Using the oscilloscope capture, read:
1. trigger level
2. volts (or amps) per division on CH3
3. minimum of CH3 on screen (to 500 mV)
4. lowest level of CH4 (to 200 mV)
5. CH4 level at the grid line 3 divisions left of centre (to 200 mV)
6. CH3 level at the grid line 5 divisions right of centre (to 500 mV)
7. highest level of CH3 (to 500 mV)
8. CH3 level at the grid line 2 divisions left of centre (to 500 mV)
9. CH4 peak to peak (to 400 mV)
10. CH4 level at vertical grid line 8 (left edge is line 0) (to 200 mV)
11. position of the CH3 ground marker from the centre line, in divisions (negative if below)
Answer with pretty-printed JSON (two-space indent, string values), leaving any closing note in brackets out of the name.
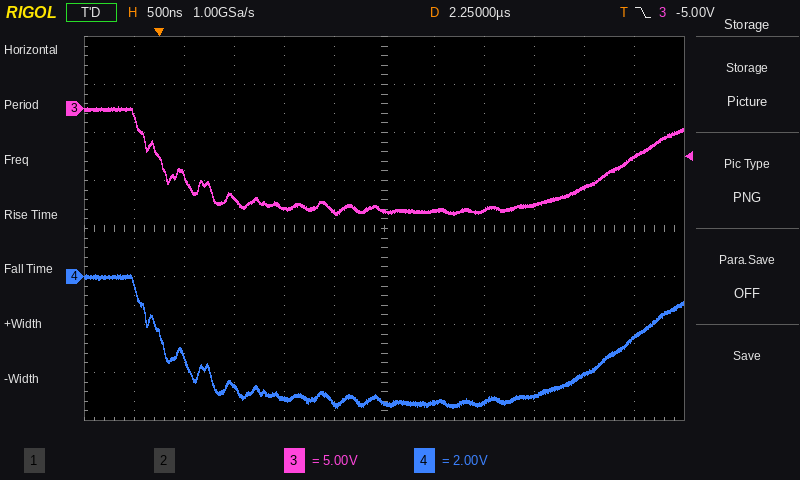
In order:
{
  "trigger level": "-5.00 V",
  "volts (or amps) per division on CH3": "5 V",
  "minimum of CH3 on screen": "-11.0 V",
  "lowest level of CH4": "-5.4 V",
  "CH4 level at the grid line 3 divisions left of centre": "-4.6 V",
  "CH3 level at the grid line 5 divisions right of centre": "-5.0 V",
  "highest level of CH3": "0.0 V",
  "CH3 level at the grid line 2 divisions left of centre": "-10.5 V",
  "CH4 peak to peak": "5.6 V",
  "CH4 level at vertical grid line 8 (left edge is line 0)": "-5.2 V",
  "position of the CH3 ground marker from the centre line, in divisions": "+2.5 div"
}
